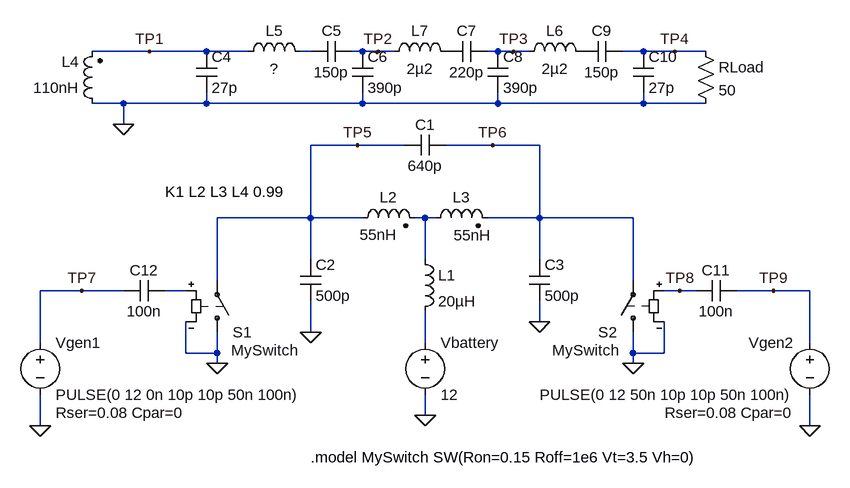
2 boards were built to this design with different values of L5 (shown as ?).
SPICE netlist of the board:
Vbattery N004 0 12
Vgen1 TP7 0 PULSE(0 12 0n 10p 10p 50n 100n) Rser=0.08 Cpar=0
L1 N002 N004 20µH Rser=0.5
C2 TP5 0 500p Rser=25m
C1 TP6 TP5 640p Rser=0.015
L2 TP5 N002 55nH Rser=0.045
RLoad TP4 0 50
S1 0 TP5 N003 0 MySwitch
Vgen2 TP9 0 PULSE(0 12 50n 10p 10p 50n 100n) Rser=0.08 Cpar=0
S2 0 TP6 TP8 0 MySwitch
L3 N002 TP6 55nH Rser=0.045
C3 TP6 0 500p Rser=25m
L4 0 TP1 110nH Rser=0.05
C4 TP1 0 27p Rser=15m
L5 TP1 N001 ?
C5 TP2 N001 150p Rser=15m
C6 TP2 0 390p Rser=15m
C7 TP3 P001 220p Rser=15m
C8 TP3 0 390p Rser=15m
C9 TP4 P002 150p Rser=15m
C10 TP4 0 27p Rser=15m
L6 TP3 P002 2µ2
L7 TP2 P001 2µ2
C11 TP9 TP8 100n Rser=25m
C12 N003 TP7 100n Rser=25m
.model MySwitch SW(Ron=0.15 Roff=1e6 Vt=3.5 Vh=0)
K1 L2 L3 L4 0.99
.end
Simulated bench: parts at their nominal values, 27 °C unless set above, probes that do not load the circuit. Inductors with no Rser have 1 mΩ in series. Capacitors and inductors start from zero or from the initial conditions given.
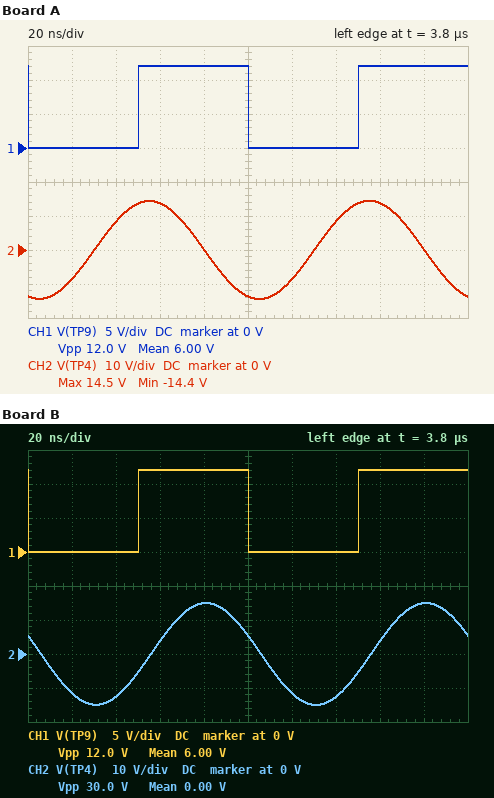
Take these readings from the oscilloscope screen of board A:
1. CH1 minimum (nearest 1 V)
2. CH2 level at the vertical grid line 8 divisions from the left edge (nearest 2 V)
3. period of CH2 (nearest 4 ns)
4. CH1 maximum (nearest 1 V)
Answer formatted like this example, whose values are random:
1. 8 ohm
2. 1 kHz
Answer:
1. 0 V
2. 14 V
3. 100 ns
4. 12 V
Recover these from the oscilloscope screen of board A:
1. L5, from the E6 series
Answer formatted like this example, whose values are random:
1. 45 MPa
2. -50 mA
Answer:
1. 1 µH
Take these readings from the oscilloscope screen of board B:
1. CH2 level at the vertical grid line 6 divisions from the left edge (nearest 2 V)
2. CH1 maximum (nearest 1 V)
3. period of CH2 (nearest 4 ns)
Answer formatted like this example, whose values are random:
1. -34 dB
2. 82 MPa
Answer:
1. -12 V
2. 12 V
3. 100 ns
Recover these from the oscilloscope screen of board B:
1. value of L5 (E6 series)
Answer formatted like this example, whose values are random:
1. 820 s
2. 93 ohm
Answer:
1. 3.3 µH
